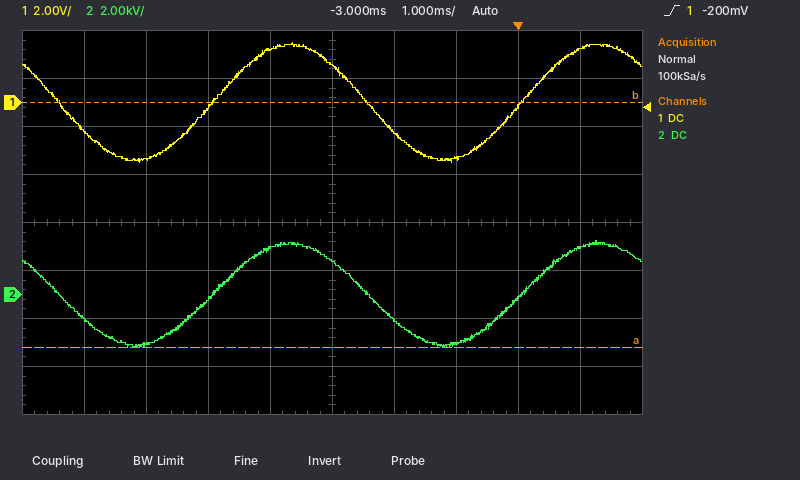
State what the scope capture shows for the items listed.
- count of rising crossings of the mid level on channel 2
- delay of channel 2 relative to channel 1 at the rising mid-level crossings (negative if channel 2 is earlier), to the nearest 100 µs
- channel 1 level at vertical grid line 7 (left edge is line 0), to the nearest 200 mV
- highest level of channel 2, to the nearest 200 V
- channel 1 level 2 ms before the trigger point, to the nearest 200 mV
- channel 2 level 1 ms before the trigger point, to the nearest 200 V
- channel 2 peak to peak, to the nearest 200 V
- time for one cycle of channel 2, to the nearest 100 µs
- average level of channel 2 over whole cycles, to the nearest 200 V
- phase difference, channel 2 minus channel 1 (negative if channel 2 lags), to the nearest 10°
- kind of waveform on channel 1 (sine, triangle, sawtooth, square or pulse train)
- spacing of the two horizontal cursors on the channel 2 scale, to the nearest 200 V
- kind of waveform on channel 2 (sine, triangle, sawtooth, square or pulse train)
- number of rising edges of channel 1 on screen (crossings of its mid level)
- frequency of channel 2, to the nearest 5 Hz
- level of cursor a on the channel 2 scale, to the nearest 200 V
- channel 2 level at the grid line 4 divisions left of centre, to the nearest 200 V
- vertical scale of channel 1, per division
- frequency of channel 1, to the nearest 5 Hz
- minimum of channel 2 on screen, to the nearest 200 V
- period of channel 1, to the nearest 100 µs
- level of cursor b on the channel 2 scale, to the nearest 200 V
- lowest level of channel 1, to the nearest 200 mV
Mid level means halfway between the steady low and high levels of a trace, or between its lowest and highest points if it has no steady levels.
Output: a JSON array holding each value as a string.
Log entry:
["2", "0.0 ms", "-2.4 V", "2.2 kV", "-1.2 V", "-2.0 kV", "4.4 kV", "5.0 ms", "0.0 kV", "0°", "sine", "10.2 kV", "sine", "2", "200 Hz", "-2.2 kV", "-1.0 kV", "2 V", "200 Hz", "-2.2 kV", "5.0 ms", "8.0 kV", "-2.4 V"]
